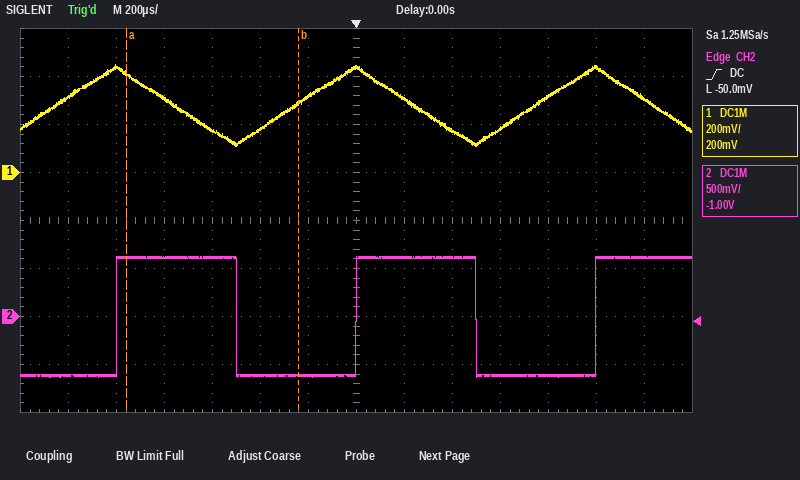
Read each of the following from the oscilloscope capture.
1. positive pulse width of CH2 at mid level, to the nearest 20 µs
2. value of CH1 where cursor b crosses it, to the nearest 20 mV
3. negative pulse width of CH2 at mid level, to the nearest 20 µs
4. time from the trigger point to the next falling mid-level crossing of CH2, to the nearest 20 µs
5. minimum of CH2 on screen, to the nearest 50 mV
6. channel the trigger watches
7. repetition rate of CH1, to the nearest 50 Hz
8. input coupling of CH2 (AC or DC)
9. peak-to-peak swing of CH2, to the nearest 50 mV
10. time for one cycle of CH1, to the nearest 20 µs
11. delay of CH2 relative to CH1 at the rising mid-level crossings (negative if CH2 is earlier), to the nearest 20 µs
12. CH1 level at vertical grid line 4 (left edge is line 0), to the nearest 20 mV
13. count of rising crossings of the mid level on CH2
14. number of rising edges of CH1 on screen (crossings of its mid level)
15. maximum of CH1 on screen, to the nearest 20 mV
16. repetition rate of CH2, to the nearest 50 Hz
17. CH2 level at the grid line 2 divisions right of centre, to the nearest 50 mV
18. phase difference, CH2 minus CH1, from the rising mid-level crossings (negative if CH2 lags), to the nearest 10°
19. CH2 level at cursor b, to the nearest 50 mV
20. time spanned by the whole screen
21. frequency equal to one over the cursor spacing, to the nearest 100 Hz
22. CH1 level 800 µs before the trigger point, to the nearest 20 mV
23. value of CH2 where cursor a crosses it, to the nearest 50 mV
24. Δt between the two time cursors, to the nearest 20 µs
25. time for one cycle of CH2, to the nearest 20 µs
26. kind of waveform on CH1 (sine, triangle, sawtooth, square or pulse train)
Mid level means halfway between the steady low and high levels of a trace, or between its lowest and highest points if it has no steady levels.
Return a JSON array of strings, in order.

["500 µs", "280 mV", "500 µs", "500 µs", "-650 mV", "CH2", "1.00 kHz", "DC", "1.25 V", "1.00 ms", "+260 µs", "180 mV", "3", "3", "440 mV", "1.00 kHz", "600 mV", "-90°", "-600 mV", "2.8 ms", "1.4 kHz", "300 mV", "600 mV", "720 µs", "1.00 ms", "triangle"]
